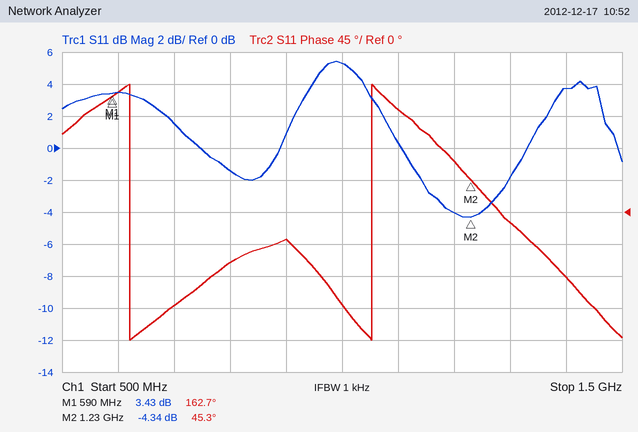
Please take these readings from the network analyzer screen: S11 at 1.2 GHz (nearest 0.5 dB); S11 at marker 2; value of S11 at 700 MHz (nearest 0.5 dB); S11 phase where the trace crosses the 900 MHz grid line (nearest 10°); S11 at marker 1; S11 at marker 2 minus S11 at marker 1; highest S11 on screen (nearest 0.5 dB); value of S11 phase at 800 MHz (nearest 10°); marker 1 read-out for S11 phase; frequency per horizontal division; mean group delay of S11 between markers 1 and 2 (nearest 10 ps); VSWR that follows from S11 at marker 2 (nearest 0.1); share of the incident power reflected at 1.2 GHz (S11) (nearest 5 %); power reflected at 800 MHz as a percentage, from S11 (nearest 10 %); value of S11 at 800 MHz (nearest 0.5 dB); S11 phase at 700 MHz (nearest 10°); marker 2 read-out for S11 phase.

-4.0 dB
-4.34 dB
1.5 dB
-40°
3.43 dB
-7.77 dB
5.5 dB
-70°
162.7°
100 MHz
510 ps
4.1
40 %
70 %
-1.5 dB
-130°
45.3°
